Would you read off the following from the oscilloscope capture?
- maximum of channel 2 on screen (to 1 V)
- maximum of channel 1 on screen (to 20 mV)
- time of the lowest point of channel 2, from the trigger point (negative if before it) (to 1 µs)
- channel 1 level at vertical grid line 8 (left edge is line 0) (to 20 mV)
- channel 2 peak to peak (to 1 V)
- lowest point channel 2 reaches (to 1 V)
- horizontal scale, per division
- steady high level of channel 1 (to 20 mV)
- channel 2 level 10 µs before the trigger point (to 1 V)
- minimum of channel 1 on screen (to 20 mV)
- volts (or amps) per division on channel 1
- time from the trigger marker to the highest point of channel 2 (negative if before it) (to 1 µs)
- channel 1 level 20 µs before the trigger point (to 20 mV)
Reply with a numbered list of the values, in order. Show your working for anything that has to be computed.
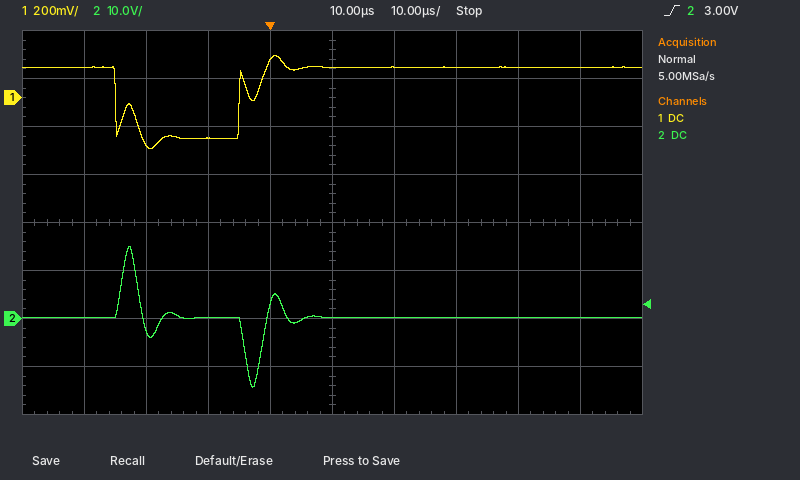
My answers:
1. 15 V
2. 180 mV
3. -3 µs
4. 120 mV
5. 15 V − (-14 V) = 29 V
6. -14 V
7. 10 µs
8. 120 mV
9. 0 V
10. -220 mV
11. 200 mV
12. -23 µs
13. -200 mV
